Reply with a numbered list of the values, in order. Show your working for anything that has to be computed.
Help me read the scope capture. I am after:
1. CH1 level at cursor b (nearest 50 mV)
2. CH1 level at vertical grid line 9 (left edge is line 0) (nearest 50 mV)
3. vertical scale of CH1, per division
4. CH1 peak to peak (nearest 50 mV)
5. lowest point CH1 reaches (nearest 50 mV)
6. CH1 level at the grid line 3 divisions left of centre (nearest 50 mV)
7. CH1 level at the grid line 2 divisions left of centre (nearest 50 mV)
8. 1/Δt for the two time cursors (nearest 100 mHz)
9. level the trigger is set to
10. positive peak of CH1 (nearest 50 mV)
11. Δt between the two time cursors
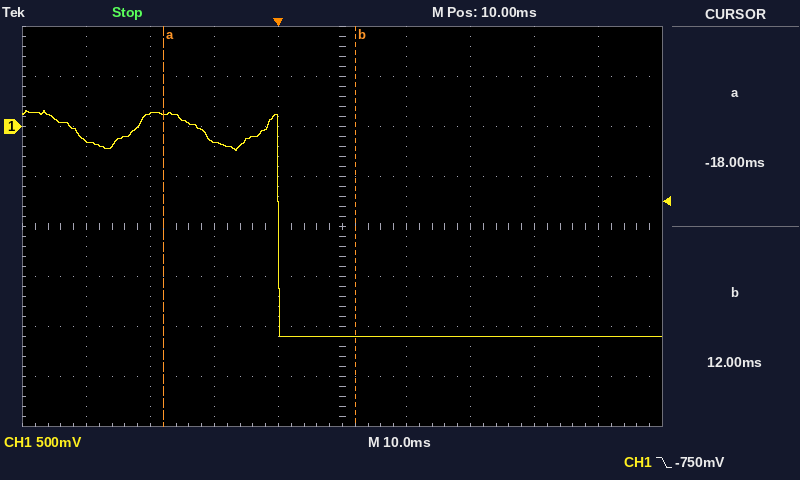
1. -2.10 V
2. -2.10 V
3. 500 mV
4. 150 mV − (-2.10 V) = 2.25 V
5. -2.10 V
6. 150 mV
7. -150 mV
8. 1 / 30 ms ≈ 33.3 Hz
9. -750 mV
10. 150 mV
11. 12 ms − (-18 ms) = 30 ms
